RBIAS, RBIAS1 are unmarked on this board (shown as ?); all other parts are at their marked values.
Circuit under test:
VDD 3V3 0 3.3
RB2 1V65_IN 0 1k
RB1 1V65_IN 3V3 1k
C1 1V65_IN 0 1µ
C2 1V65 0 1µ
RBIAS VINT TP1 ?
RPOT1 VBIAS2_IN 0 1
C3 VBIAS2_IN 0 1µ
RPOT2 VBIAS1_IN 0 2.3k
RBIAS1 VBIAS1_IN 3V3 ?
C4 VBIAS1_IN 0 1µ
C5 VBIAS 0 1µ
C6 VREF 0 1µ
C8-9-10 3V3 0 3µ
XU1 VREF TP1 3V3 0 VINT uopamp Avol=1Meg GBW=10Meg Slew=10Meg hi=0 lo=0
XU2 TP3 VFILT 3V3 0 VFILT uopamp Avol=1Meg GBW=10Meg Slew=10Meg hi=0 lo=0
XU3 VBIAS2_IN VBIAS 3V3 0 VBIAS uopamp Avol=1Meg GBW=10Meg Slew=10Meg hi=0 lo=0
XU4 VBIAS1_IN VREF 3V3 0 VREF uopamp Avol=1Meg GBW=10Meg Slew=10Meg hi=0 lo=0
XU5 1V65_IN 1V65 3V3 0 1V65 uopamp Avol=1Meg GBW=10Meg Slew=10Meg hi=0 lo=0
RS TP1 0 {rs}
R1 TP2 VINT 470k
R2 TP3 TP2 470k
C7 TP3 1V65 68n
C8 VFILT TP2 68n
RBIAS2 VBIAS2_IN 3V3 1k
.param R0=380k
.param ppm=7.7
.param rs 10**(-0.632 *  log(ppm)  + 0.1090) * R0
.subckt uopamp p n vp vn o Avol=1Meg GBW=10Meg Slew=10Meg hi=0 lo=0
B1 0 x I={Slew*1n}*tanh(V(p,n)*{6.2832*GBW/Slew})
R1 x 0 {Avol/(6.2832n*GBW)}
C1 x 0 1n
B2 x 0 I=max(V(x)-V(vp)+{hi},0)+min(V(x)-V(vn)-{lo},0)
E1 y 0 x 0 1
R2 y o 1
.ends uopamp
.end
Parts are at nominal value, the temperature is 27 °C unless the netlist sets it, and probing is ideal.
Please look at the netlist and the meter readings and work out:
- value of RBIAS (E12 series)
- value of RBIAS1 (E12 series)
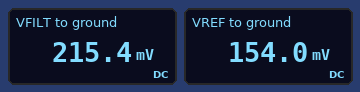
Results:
10 kΩ
47 kΩ
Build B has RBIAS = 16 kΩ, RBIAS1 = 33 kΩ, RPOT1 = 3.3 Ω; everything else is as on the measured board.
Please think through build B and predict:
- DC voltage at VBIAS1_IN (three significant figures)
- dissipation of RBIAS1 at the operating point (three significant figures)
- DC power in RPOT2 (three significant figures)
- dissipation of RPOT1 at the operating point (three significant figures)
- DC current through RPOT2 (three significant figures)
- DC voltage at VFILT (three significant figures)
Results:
215 mV
288 µW
20.1 µW
35.7 µW
93.5 µA
352 mV
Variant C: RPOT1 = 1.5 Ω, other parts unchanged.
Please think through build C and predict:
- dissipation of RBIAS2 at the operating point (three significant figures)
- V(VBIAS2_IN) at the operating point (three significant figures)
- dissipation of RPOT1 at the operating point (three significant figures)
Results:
10.9 mW
4.94 mV
16.3 µW
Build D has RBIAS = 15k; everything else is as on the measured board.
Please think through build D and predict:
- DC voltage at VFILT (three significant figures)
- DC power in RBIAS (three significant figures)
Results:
246 mV
567 nW
